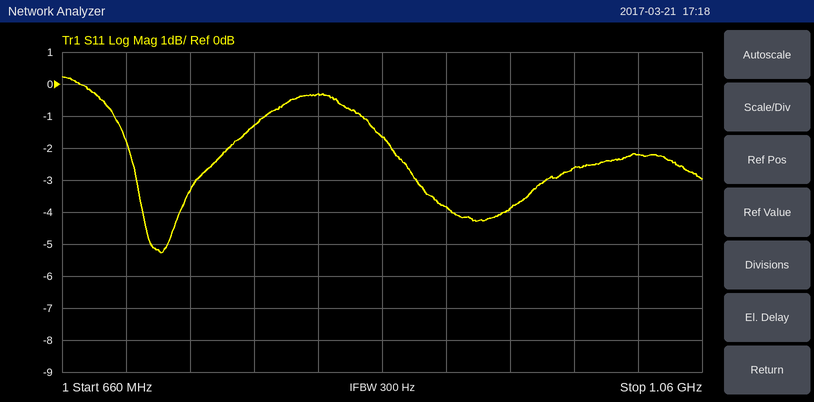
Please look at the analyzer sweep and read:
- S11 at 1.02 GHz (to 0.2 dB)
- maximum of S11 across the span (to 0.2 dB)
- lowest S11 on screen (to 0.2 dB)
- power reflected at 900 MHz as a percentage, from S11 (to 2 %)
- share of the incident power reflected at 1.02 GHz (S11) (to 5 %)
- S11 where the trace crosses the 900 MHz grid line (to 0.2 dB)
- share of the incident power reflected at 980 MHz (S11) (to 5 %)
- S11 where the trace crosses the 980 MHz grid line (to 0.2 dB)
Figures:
-2.2 dB
0.2 dB
-5.2 dB
42 %
60 %
-3.8 dB
55 %
-2.6 dB
